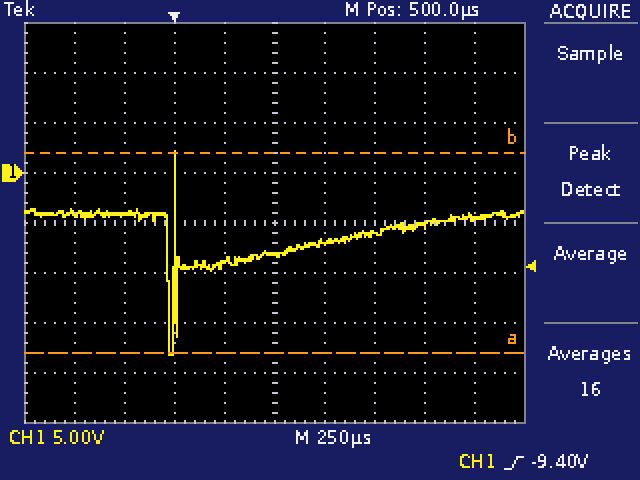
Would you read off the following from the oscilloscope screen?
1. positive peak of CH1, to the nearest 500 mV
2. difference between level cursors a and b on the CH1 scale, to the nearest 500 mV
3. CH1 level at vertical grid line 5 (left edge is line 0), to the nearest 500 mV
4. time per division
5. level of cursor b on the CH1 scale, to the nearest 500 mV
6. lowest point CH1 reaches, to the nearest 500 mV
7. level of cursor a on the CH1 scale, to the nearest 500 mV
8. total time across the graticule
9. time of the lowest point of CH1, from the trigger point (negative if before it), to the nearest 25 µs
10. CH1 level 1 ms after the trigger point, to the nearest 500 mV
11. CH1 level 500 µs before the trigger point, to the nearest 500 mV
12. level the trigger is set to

2.0 V
20.0 V
-8.0 V
250 µs
2.0 V
-18.0 V
-18.0 V
2.5 ms
-25 µs
-6.0 V
-4.0 V
-9.40 V
